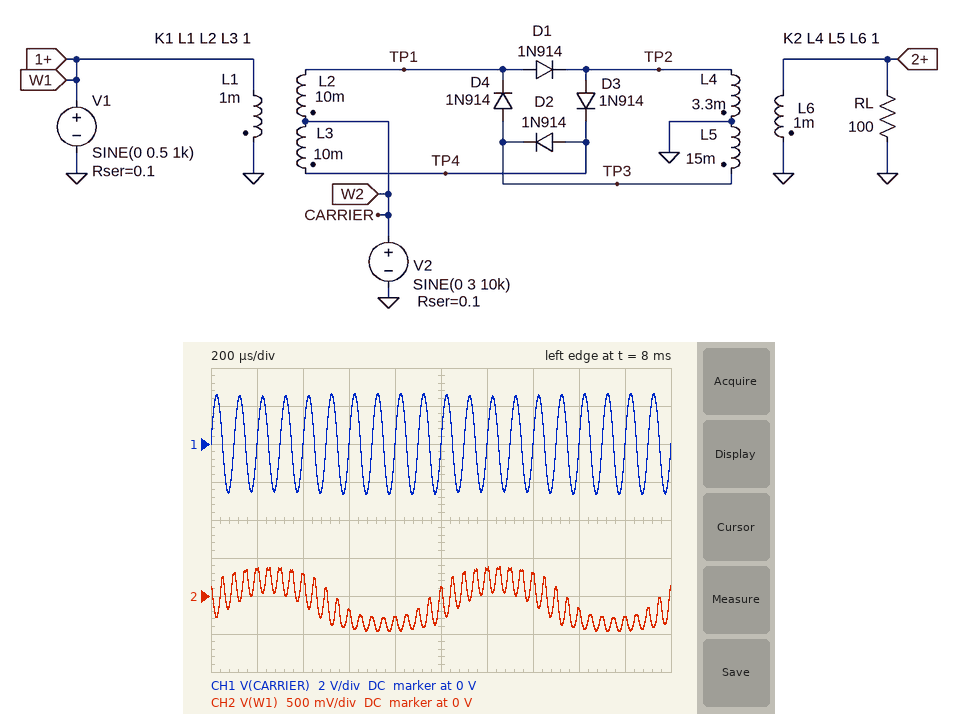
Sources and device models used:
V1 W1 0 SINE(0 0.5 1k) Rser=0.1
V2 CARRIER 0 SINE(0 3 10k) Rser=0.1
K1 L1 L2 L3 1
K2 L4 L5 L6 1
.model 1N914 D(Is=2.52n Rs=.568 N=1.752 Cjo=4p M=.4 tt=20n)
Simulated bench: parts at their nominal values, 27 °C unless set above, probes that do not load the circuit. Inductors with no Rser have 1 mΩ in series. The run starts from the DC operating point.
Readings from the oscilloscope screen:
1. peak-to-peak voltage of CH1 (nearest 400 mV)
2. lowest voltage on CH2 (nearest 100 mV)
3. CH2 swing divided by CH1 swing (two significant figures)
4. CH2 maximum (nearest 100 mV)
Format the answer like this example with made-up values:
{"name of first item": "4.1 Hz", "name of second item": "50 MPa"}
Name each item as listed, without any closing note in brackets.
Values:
{"peak-to-peak voltage of CH1": "5.2 V", "lowest voltage on CH2": "-500 mV", "CH2 swing divided by CH1 swing": "0.16", "CH2 maximum": "400 mV"}
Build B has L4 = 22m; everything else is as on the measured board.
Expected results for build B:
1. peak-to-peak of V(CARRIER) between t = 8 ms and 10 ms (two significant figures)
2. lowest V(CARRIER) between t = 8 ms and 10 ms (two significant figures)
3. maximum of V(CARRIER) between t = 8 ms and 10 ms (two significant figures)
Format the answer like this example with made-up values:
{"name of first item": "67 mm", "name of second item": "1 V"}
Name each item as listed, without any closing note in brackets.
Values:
{"peak-to-peak of V(CARRIER) between t = 8 ms and 10 ms": "5.0 V", "lowest V(CARRIER) between t = 8 ms and 10 ms": "-2.5 V", "maximum of V(CARRIER) between t = 8 ms and 10 ms": "2.5 V"}
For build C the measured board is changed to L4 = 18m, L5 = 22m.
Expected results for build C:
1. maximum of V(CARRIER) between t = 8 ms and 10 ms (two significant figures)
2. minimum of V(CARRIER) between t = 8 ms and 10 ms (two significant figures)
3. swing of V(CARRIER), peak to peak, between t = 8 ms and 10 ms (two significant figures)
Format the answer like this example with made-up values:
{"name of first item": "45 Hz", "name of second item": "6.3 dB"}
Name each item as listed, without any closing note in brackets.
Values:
{"maximum of V(CARRIER) between t = 8 ms and 10 ms": "2.5 V", "minimum of V(CARRIER) between t = 8 ms and 10 ms": "-2.5 V", "swing of V(CARRIER), peak to peak, between t = 8 ms and 10 ms": "5.0 V"}
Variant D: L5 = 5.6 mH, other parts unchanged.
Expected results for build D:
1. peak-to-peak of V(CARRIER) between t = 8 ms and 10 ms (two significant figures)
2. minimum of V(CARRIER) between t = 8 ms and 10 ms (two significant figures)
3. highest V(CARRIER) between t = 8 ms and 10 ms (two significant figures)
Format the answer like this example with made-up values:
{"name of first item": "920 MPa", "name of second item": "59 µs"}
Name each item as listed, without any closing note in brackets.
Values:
{"peak-to-peak of V(CARRIER) between t = 8 ms and 10 ms": "5.1 V", "minimum of V(CARRIER) between t = 8 ms and 10 ms": "-2.5 V", "highest V(CARRIER) between t = 8 ms and 10 ms": "2.5 V"}
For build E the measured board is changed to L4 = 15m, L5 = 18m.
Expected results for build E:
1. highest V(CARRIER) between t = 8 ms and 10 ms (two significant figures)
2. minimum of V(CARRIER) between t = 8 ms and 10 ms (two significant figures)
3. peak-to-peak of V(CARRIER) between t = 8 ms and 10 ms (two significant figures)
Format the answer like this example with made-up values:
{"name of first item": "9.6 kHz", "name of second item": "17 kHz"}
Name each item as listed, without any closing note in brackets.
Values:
{"highest V(CARRIER) between t = 8 ms and 10 ms": "2.5 V", "minimum of V(CARRIER) between t = 8 ms and 10 ms": "-2.5 V", "peak-to-peak of V(CARRIER) between t = 8 ms and 10 ms": "5.0 V"}
